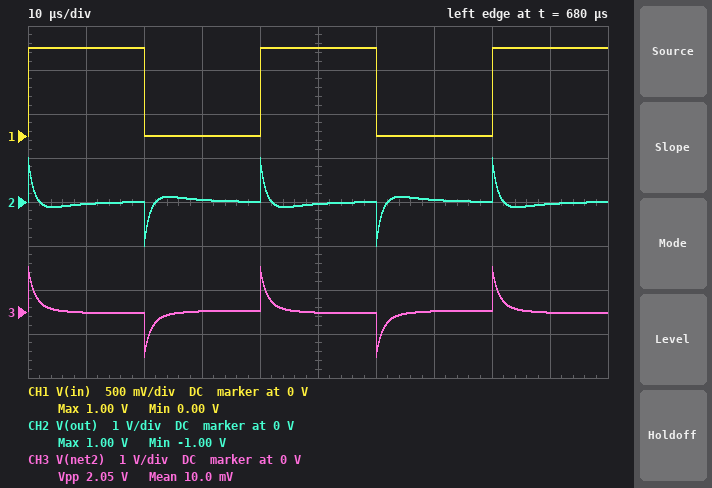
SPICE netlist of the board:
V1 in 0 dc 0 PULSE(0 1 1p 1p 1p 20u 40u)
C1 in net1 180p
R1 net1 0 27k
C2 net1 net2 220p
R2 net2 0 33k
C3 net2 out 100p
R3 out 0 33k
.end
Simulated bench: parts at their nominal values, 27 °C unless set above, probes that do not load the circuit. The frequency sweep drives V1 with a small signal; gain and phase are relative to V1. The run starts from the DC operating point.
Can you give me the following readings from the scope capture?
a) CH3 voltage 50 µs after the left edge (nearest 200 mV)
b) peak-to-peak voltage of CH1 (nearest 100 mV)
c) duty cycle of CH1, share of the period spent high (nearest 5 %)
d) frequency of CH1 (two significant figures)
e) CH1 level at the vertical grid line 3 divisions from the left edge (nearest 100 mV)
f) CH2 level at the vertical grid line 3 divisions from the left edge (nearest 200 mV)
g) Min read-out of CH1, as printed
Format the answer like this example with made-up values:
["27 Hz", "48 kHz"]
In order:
["0 V", "1.0 V", "50 %", "25 kHz", "0 V", "0 V", "0.00 V"]
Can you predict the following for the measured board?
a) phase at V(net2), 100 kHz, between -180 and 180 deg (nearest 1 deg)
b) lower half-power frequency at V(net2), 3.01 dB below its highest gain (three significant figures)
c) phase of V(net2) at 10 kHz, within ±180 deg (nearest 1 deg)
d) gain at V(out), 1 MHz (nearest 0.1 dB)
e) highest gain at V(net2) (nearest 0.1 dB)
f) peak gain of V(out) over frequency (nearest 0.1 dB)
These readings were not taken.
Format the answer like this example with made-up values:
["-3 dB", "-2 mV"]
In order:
["49 deg", "132 kHz", "119 deg", "-0.1 dB", "0 dB", "0 dB"]
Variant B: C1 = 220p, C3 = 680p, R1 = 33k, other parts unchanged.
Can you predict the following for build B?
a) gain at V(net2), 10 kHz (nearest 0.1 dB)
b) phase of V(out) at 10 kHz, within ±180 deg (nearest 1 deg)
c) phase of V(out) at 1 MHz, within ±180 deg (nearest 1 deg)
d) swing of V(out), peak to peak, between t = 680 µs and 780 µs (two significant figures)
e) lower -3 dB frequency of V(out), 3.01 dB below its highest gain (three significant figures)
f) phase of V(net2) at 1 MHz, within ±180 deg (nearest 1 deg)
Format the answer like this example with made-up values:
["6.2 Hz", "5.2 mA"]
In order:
["-22.1 dB", "148 deg", "7 deg", "2.1 V", "104 kHz", "6 deg"]
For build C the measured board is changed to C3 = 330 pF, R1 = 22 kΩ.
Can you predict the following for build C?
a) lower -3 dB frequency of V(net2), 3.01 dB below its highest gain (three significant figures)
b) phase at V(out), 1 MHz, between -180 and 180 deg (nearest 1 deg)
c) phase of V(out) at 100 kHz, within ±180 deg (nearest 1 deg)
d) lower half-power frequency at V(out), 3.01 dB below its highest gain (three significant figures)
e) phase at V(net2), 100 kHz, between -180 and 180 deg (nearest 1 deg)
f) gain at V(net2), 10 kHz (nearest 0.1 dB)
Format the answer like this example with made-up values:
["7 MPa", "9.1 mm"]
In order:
["130 kHz", "9 deg", "65 deg", "132 kHz", "57 deg", "-24.5 dB"]
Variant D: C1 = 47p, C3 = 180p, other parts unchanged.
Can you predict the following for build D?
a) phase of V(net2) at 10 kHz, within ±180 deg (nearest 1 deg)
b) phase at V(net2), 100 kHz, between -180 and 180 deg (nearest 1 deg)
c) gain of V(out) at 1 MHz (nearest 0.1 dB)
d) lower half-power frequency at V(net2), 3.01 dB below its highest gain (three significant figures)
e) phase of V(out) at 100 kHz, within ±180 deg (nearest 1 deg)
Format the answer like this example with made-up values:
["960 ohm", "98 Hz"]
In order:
["126 deg", "78 deg", "-0.6 dB", "369 kHz", "93 deg"]
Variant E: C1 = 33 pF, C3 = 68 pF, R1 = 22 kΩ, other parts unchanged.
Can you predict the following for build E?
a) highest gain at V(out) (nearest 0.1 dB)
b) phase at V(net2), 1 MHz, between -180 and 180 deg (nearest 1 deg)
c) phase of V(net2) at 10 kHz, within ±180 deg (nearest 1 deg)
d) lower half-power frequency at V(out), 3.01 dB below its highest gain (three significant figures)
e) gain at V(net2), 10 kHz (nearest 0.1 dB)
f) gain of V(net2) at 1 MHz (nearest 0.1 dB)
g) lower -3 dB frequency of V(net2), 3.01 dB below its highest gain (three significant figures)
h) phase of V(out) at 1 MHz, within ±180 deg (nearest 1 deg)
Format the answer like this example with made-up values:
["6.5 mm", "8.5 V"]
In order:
["0 dB", "29 deg", "135 deg", "567 kHz", "-36.2 dB", "-1.2 dB", "558 kHz", "33 deg"]
